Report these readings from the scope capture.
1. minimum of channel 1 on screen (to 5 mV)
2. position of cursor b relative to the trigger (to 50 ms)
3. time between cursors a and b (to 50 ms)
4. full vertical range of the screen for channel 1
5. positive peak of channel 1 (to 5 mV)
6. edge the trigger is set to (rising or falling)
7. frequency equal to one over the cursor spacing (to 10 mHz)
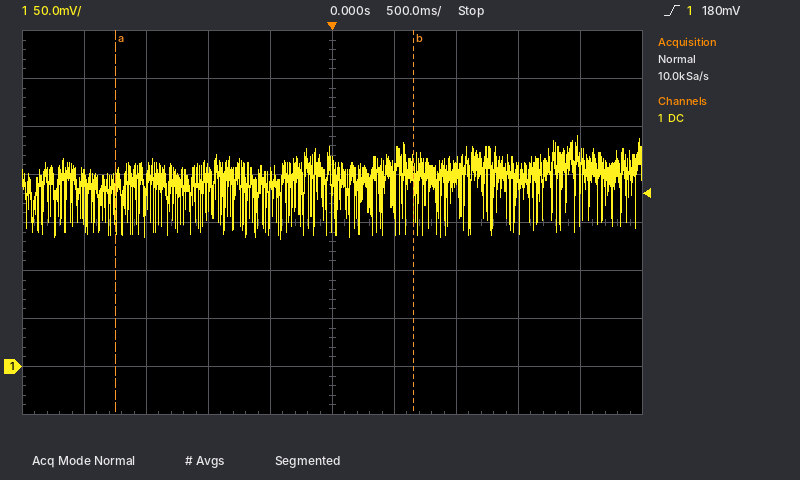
135 mV
+650 ms
2.40 s
400 mV
240 mV
rising
420 mHz
